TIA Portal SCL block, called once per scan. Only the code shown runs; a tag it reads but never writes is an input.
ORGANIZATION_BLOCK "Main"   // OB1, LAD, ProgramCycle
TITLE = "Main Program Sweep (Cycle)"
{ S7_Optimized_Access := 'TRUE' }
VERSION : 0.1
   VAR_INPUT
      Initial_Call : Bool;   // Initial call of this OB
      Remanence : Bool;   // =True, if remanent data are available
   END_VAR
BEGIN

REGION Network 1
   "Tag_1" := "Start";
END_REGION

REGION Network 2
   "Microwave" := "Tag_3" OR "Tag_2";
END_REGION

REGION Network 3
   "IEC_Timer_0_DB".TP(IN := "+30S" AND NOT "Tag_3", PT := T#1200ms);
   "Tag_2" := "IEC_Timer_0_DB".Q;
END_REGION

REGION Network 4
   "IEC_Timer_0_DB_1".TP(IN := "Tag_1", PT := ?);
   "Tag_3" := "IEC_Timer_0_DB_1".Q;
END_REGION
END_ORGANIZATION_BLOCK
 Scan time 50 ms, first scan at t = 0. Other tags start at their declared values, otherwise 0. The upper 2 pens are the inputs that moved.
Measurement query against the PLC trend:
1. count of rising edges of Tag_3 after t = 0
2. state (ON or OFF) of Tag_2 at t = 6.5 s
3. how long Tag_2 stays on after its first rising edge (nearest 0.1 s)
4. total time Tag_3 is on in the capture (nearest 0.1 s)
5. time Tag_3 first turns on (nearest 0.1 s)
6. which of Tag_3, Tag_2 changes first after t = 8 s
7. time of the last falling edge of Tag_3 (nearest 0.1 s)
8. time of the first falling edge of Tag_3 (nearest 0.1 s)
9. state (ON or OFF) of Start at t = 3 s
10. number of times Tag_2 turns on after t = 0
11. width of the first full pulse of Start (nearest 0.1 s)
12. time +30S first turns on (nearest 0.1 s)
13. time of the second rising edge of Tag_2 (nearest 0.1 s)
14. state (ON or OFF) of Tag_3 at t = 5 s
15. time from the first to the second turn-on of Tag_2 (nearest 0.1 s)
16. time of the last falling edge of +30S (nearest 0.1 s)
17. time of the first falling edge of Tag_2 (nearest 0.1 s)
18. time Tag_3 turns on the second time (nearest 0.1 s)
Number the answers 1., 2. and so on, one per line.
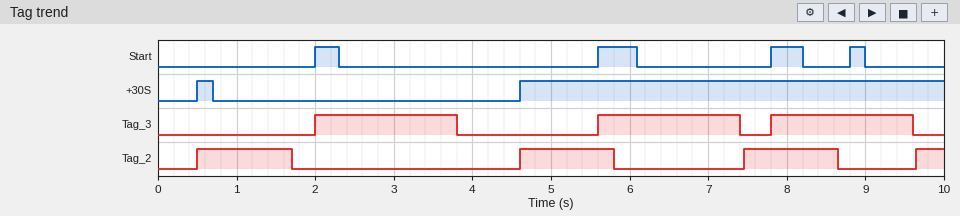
1. 3
2. OFF
3. 1.2 s
4. 5.4 s
5. 2.0 s
6. Tag_2
7. 9.6 s
8. 3.8 s
9. OFF
10. 4
11. 0.3 s
12. 0.5 s
13. 4.6 s
14. OFF
15. 4.1 s
16. 0.7 s
17. 1.7 s
18. 5.6 s
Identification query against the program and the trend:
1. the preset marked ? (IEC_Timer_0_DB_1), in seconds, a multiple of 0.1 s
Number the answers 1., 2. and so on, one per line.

1. 1.8 s
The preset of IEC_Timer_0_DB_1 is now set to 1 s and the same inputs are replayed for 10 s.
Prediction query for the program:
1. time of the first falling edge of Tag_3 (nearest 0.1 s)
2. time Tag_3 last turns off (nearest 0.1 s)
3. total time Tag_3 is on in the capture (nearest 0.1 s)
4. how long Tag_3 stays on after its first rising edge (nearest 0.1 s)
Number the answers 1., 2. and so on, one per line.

1. 3.0 s
2. 8.8 s
3. 3.0 s
4. 1.0 s
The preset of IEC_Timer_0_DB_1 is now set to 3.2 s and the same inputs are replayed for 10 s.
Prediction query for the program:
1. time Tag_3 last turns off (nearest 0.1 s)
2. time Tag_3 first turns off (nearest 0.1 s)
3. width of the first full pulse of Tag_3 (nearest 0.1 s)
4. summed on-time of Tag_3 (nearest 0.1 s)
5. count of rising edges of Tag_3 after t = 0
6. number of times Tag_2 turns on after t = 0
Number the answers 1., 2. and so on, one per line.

1. 8.8 s
2. 5.2 s
3. 3.2 s
4. 6.4 s
5. 2
6. 3
